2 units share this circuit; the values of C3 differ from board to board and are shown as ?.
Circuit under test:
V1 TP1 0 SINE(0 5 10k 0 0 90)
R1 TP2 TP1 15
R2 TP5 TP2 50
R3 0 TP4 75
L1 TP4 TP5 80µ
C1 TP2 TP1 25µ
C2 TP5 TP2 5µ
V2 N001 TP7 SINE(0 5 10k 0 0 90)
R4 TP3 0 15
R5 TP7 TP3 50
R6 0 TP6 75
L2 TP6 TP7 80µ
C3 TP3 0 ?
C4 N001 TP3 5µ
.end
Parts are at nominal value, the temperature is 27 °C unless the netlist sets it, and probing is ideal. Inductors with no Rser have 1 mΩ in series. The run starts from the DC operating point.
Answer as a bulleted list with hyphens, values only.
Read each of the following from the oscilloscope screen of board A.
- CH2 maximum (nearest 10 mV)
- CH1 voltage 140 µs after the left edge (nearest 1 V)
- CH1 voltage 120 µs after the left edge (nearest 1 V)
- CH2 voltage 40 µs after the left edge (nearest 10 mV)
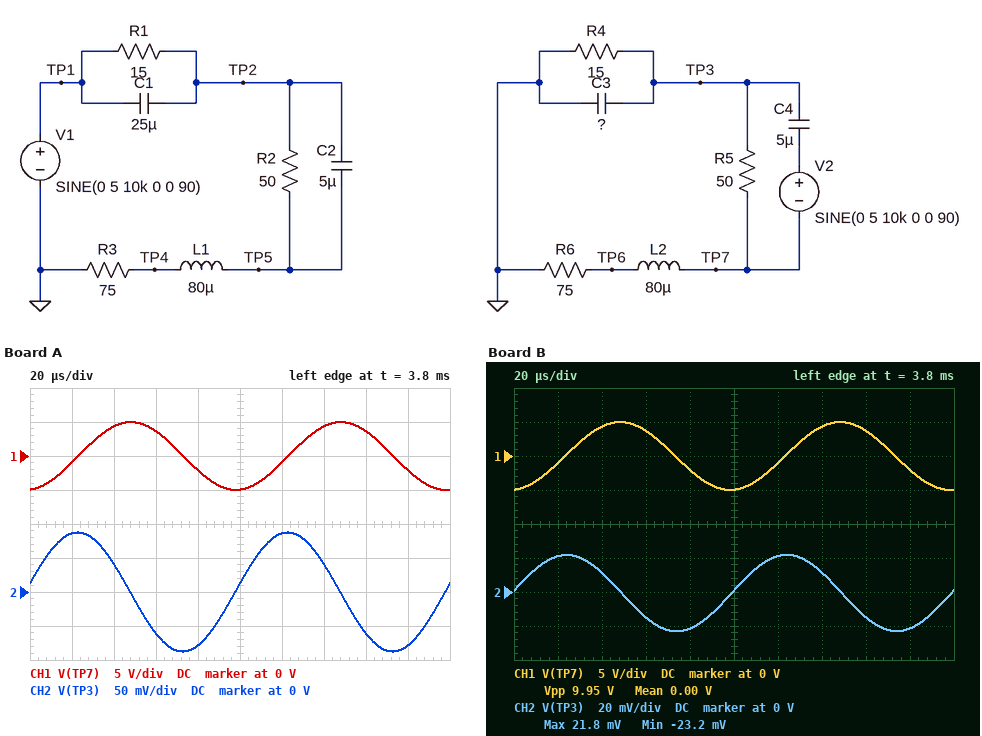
- 90 mV
- 4 V
- -1 V
- 40 mV
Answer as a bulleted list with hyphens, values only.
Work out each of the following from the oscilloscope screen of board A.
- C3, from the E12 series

- 12 µF
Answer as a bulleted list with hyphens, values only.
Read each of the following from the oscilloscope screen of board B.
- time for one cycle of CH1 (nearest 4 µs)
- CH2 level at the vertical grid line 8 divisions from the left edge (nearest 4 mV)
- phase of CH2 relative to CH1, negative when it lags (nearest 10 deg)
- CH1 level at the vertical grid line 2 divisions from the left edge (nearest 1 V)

- 100 µs
- -16 mV
- 90 deg
- 4 V
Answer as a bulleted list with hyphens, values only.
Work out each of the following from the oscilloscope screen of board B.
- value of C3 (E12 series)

- 47 µF
